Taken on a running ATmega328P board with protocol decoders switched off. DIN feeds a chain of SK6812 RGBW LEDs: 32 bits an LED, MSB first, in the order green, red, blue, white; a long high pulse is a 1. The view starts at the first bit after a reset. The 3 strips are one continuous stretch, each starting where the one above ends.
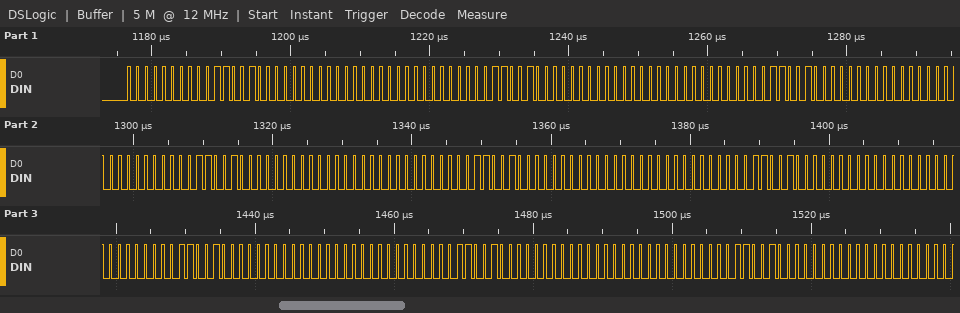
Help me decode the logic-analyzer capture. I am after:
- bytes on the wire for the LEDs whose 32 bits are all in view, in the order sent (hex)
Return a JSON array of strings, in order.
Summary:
["00 32 00 00 00 32 00 00 00 32 00 00 00 32 00 00 00 32 00 00 00 32 00 00 00 32 00 00 00 32 00 00 00 32 00 00"]
